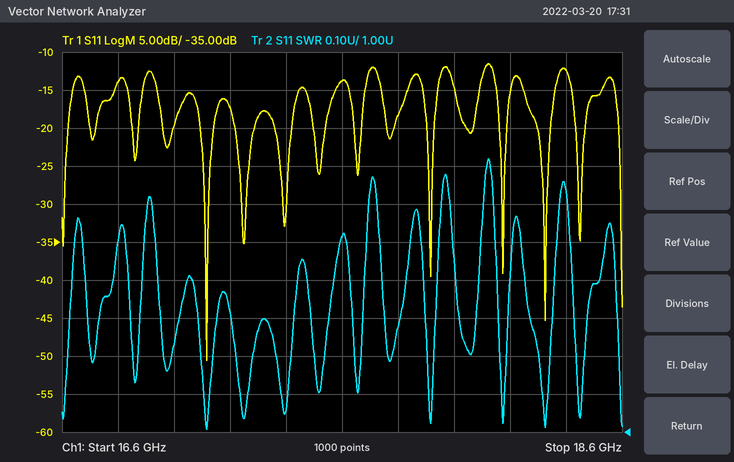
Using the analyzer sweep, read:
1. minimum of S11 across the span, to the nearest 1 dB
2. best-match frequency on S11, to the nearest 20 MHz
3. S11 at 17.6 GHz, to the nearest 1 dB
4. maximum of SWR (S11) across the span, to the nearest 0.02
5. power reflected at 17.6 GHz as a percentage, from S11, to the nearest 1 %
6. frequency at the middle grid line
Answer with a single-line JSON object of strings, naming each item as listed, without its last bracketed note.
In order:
{"minimum of S11 across the span, to the nearest 1 dB": "-51 dB", "best-match frequency on S11, to the nearest 20 MHz": "17.12 GHz", "S11 at 17.6 GHz, to the nearest 1 dB": "-14 dB", "maximum of SWR (S11) across the span, to the nearest 0.02": "1.72", "power reflected at 17.6 GHz as a percentage, from S11, to the nearest 1 %": "4 %", "frequency at the middle grid line": "17.6 GHz"}
